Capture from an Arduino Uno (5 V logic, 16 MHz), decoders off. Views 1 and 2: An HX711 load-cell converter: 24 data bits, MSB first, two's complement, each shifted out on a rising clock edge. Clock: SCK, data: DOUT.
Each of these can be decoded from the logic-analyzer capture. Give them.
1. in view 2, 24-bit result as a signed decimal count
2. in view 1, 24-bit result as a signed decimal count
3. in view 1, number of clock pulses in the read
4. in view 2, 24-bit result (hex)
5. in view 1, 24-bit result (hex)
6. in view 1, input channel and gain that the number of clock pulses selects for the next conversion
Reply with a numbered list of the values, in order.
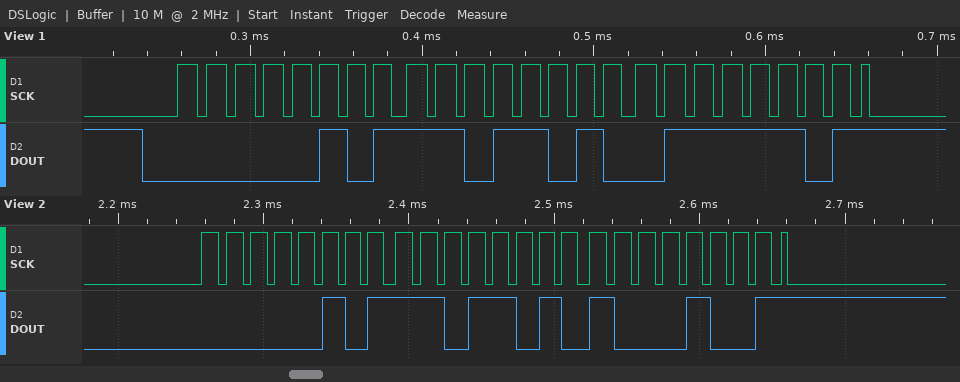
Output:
1. 383625
2. 383613
3. 25
4. 0x05DA89
5. 0x05DA7D
6. channel A, gain 128
